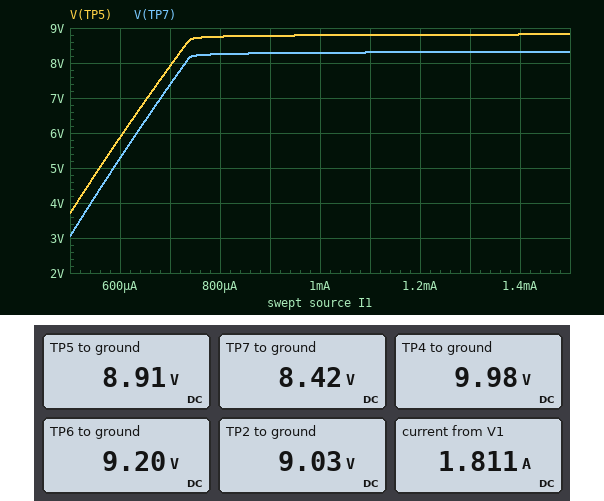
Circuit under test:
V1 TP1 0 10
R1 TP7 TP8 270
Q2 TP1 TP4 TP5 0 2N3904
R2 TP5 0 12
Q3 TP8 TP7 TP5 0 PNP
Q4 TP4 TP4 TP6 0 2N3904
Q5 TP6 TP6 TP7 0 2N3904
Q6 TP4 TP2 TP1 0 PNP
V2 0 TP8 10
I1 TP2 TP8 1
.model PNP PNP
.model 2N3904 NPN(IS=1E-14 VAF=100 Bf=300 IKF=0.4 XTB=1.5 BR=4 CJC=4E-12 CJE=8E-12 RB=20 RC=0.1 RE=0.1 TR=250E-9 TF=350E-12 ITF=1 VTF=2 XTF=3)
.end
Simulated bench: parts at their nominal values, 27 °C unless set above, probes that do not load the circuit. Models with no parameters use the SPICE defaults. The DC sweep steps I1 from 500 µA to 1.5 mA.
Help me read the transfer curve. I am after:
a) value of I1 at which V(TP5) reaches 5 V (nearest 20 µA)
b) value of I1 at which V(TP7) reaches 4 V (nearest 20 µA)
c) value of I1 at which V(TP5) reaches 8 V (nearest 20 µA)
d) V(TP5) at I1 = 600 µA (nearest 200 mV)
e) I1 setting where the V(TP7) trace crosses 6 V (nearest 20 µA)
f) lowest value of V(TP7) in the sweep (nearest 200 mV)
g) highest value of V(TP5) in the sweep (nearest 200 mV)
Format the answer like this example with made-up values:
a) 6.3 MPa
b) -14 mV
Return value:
a) 560 µA
b) 540 µA
c) 700 µA
d) 5.8 V
e) 640 µA
f) 3.0 V
g) 8.8 V
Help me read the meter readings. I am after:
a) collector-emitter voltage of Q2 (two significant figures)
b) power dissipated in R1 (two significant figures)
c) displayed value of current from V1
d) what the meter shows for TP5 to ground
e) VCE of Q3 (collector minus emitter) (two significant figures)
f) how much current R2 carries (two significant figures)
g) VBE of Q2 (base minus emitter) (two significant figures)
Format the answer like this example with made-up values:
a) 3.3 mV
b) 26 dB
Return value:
a) 1.1 V
b) 1.3 W
c) 1.811 A
d) 8.91 V
e) -19 V
f) 740 mA
g) 1.1 V
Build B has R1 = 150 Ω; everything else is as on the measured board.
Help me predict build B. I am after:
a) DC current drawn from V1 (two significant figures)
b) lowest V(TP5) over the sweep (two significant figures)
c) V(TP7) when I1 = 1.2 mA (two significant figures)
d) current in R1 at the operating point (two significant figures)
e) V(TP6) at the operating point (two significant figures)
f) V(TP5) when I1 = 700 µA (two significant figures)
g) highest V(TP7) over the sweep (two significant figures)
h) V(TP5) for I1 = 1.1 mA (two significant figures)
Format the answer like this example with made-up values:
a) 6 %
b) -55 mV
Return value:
a) 1.9 A
b) -1.4 V
c) 7.2 V
d) 120 mA
e) 9.2 V
f) 1.2 V
g) 8.2 V
h) 6.5 V
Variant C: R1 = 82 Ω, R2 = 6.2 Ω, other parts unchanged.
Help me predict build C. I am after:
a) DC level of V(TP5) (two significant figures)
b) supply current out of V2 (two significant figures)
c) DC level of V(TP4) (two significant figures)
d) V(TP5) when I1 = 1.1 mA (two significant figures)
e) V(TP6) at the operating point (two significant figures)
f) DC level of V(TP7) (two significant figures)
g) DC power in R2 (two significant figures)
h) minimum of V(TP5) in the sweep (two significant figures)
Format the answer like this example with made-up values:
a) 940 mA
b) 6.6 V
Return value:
a) 8.6 V
b) 1.2 A
c) 10 V
d) -88 mV
e) 9.1 V
f) 8.3 V
g) 12 W
h) -4.4 V
